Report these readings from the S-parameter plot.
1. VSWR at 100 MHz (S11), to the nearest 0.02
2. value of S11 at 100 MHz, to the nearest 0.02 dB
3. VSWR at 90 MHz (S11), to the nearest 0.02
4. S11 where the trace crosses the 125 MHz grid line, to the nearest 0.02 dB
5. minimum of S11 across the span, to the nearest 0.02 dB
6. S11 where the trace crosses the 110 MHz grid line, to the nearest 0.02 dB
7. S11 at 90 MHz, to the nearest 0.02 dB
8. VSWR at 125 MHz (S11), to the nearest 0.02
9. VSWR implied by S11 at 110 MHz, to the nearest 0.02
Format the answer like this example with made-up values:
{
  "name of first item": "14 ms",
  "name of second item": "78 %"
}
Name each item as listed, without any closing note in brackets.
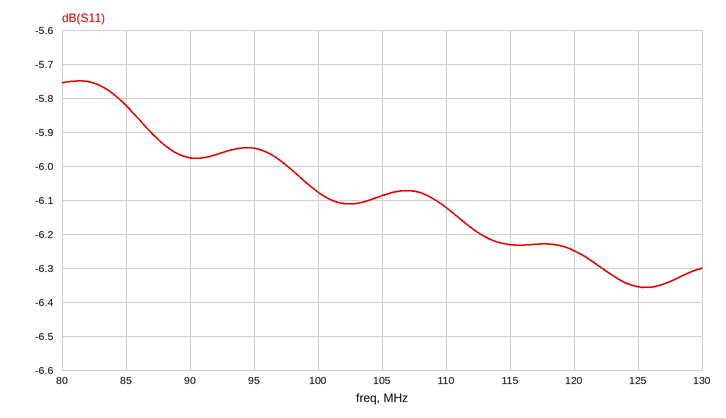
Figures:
{
  "VSWR at 100 MHz (S11), to the nearest 0.02": "2.98",
  "value of S11 at 100 MHz, to the nearest 0.02 dB": "-6.08 dB",
  "VSWR at 90 MHz (S11), to the nearest 0.02": "3.02",
  "S11 where the trace crosses the 125 MHz grid line, to the nearest 0.02 dB": "-6.36 dB",
  "minimum of S11 across the span, to the nearest 0.02 dB": "-6.36 dB",
  "S11 where the trace crosses the 110 MHz grid line, to the nearest 0.02 dB": "-6.12 dB",
  "S11 at 90 MHz, to the nearest 0.02 dB": "-5.98 dB",
  "VSWR at 125 MHz (S11), to the nearest 0.02": "2.86",
  "VSWR implied by S11 at 110 MHz, to the nearest 0.02": "2.96"
}
